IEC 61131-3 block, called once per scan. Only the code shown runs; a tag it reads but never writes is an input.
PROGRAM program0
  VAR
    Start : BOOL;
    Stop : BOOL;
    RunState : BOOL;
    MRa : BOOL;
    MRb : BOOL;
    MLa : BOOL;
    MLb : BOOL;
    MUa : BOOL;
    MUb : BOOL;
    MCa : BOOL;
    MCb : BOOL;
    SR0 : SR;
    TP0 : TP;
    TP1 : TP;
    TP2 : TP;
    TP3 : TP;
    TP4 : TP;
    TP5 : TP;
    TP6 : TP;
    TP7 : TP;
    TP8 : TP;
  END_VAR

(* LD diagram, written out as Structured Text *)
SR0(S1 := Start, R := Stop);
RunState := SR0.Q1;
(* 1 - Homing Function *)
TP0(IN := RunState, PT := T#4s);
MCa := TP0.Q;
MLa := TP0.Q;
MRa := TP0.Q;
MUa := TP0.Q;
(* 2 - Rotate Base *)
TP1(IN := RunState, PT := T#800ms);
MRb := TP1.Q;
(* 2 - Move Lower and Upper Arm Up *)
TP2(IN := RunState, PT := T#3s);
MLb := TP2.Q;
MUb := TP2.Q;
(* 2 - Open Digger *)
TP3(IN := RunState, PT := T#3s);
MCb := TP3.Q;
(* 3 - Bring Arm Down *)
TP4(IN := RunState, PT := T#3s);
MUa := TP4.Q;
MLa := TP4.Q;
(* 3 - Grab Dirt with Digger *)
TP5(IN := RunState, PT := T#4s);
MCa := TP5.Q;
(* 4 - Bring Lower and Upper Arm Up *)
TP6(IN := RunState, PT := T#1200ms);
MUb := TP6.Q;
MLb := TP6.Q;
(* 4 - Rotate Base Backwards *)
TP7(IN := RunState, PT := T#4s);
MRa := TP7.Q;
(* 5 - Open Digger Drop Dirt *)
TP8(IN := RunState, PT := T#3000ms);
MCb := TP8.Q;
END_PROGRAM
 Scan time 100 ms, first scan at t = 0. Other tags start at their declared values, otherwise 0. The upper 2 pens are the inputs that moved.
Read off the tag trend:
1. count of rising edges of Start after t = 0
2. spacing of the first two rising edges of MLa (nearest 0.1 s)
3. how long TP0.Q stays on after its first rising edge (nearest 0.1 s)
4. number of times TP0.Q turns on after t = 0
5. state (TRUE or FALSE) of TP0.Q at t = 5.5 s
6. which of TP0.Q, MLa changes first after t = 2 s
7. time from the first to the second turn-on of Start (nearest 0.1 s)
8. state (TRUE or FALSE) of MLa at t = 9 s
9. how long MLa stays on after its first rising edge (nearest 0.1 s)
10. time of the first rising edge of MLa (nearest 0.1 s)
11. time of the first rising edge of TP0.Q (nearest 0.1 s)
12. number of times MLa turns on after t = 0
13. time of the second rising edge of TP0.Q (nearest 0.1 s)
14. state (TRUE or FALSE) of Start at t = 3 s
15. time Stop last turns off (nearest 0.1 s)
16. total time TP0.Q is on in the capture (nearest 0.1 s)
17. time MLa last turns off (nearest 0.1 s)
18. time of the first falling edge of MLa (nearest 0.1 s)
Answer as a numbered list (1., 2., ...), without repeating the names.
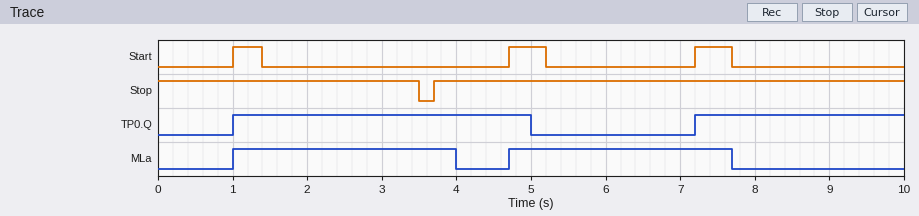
1. 3
2. 3.7 s
3. 4.0 s
4. 2
5. FALSE
6. MLa
7. 3.7 s
8. FALSE
9. 3.0 s
10. 1.0 s
11. 1.0 s
12. 2
13. 7.2 s
14. FALSE
15. 3.5 s
16. 6.8 s
17. 7.7 s
18. 4.0 s
